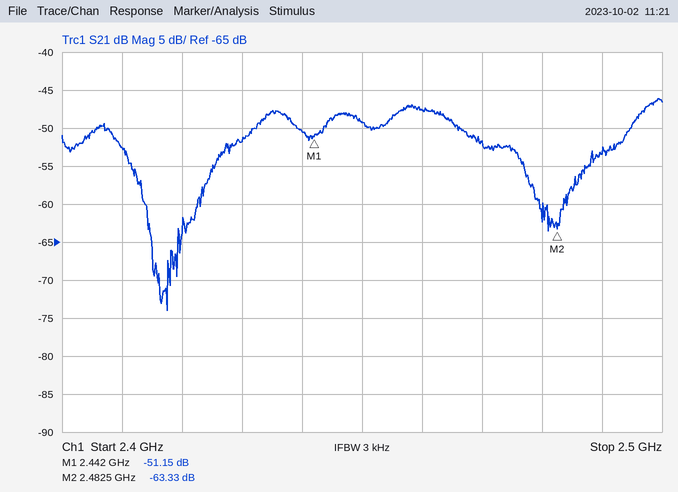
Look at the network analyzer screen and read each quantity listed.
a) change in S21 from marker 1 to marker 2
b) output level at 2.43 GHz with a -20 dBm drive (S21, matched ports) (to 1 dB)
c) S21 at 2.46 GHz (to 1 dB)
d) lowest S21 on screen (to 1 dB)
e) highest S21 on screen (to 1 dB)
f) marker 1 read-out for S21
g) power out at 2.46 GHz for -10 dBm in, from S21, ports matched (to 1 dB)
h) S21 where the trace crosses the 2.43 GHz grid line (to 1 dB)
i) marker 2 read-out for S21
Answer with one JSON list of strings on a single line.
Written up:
["-12.18 dB", "-72 dBm", "-48 dB", "-74 dB", "-46 dB", "-51.15 dB", "-58 dBm", "-52 dB", "-63.33 dB"]
